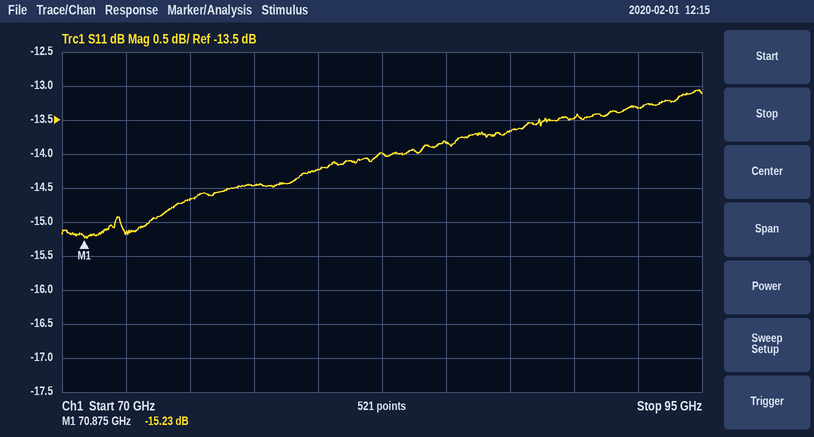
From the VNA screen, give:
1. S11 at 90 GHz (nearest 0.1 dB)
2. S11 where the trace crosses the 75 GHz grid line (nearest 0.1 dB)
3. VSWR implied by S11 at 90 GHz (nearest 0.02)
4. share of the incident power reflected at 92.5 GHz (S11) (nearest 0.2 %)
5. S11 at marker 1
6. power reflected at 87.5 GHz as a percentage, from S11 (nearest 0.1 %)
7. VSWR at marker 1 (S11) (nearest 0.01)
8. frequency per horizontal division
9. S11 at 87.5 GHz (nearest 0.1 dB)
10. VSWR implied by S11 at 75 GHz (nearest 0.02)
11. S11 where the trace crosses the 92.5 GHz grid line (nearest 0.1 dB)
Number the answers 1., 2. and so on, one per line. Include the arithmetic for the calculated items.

1. -13.5 dB
2. -14.7 dB
3. |Γ| = 10^(-13.5/20) = 0.2113; VSWR = (1 + 0.2113)/(1 − 0.2113) ≈ 1.54
4. 10^(-13.3/10) ≈ 4.68 %, so 4.6 % to the nearest 0.2 %
5. -15.23 dB
6. 10^(-13.7/10) ≈ 4.3 %
7. (1 + 0.1732)/(1 − 0.1732) ≈ 1.42
8. 2.5 GHz
9. -13.7 dB
10. |Γ| = 10^(-14.7/20) = 0.1841; VSWR = (1 + 0.1841)/(1 − 0.1841) ≈ 1.45, so 1.46 to the nearest 0.02
11. -13.3 dB
